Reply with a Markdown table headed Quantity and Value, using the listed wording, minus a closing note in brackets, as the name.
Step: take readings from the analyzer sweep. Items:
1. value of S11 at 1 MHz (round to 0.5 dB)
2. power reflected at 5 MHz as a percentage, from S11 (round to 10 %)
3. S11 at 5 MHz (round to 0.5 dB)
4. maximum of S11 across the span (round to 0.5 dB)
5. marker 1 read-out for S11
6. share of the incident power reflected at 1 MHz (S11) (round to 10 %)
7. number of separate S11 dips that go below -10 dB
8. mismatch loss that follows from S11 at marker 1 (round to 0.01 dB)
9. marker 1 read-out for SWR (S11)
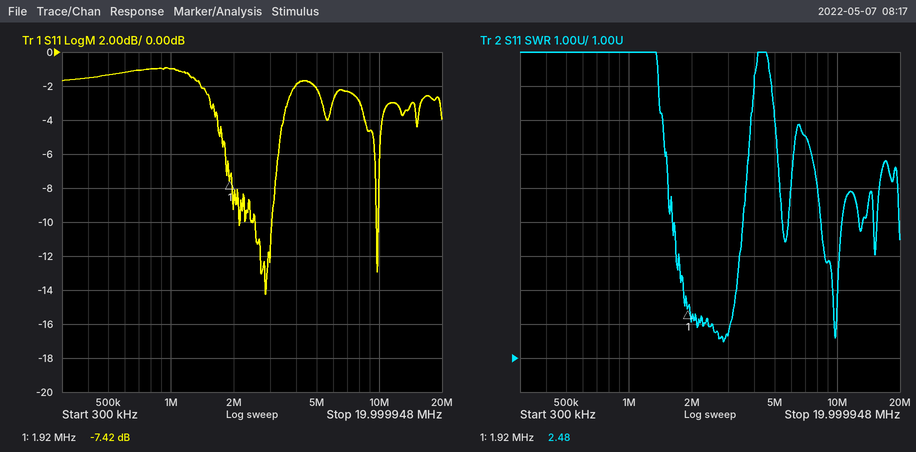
| Quantity | Value |
|---|---|
| value of S11 at 1 MHz | -1.0 dB |
| power reflected at 5 MHz as a percentage, from S11 | 60 % |
| S11 at 5 MHz | -2.0 dB |
| maximum of S11 across the span | -1.0 dB |
| marker 1 read-out for S11 | -7.42 dB |
| share of the incident power reflected at 1 MHz (S11) | 80 % |
| number of separate S11 dips that go below -10 dB | 2 |
| mismatch loss that follows from S11 at marker 1 | 0.87 dB |
| marker 1 read-out for SWR | 2.48 |
